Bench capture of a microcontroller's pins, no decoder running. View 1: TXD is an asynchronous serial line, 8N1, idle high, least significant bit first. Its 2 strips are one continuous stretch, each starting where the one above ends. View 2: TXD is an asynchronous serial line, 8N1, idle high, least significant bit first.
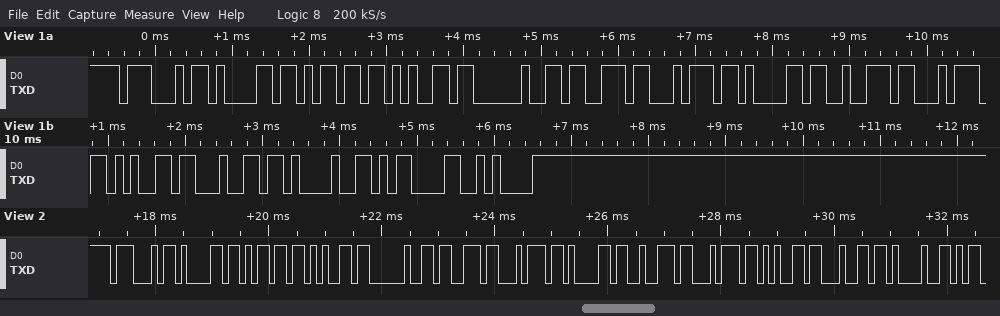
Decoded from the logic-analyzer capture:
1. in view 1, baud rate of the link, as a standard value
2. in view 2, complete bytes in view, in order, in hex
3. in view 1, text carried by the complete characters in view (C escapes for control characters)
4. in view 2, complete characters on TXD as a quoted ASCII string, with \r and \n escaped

9600 baud
0x47 0x61 0x6D 0x65 0x20 0x73 0x74 0x61 0x72 0x74 0x65 0x64 0x21
"Game started!\r\n"
"Game started!"
